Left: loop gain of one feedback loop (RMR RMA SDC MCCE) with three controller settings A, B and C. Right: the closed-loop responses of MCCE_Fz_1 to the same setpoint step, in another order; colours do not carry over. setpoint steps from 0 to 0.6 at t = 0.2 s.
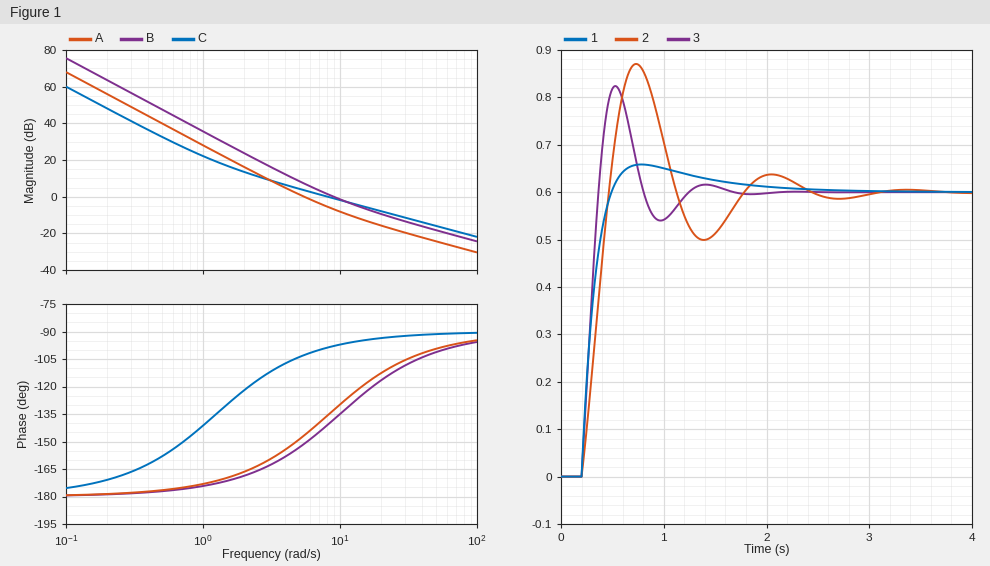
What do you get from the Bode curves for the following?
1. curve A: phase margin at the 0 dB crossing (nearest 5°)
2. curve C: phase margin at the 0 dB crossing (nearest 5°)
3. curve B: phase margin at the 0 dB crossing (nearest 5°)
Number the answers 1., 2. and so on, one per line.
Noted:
1. 35°
2. 80°
3. 40°
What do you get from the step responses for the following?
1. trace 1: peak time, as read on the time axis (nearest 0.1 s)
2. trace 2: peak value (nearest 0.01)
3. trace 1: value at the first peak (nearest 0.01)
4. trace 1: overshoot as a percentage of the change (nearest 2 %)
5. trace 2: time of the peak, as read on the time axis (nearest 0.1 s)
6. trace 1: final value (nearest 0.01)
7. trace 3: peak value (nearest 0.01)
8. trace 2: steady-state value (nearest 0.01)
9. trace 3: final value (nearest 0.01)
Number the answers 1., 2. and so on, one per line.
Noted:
1. 0.8 s
2. 0.87
3. 0.66
4. 10 %
5. 0.7 s
6. 0.60
7. 0.82
8. 0.60
9. 0.60
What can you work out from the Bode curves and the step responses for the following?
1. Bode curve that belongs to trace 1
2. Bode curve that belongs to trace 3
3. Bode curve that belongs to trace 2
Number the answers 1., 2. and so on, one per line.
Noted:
1. C
2. B
3. A
